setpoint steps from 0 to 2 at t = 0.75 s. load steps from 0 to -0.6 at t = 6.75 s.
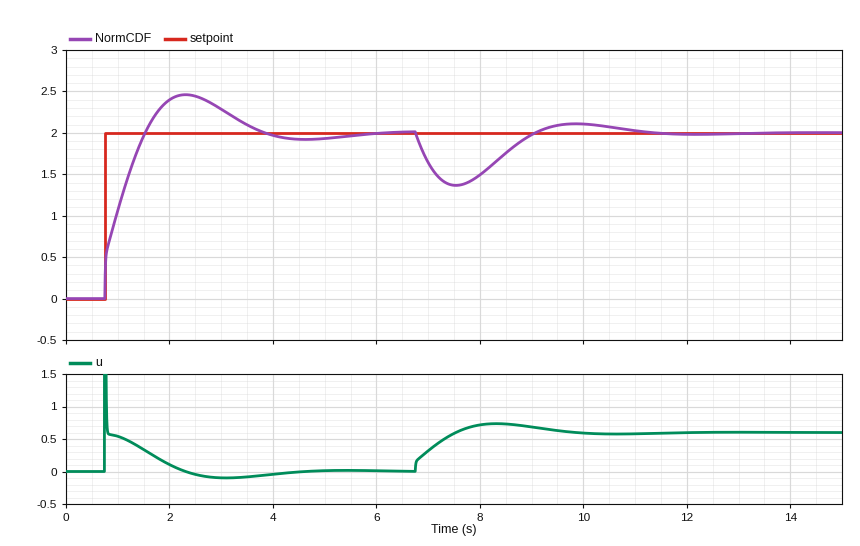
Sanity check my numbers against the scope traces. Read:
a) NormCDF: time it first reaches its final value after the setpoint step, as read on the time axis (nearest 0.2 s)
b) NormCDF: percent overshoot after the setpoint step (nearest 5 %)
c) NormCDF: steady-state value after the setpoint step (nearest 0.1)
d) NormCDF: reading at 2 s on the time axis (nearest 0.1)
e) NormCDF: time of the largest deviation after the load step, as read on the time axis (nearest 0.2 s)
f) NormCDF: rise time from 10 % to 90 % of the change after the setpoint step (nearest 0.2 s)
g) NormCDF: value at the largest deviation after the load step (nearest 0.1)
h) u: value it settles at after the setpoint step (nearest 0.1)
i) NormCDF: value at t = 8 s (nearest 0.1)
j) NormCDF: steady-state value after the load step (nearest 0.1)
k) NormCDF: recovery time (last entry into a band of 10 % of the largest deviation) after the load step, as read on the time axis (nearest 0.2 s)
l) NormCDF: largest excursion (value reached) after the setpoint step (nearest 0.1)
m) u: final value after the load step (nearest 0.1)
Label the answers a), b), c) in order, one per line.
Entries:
a) 1.6 s
b) 25 %
c) 2.0
d) 2.4
e) 7.6 s
f) 0.6 s
g) 1.4
h) 0.0
i) 1.5
j) 2.0
k) 10.6 s
l) 2.5
m) 0.6
